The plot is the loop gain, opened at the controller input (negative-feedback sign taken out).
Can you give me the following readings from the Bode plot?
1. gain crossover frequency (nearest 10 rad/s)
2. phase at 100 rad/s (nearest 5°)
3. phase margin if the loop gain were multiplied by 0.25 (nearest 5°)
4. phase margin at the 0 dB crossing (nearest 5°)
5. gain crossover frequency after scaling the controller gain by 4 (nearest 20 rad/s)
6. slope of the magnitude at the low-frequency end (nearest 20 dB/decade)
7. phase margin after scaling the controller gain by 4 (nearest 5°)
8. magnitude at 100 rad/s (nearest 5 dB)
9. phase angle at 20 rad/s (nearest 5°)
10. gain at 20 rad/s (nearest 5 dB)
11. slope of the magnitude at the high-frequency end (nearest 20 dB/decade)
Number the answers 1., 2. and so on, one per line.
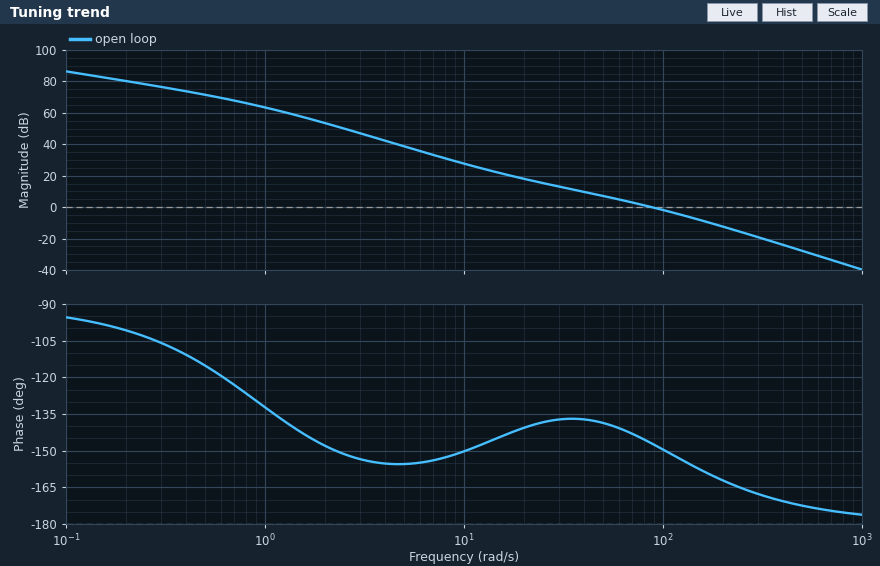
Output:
1. 90 rad/s
2. -150°
3. 45°
4. 35°
5. 200 rad/s
6. -20 dB/decade
7. 20°
8. 0 dB
9. -140°
10. 20 dB
11. -40 dB/decade
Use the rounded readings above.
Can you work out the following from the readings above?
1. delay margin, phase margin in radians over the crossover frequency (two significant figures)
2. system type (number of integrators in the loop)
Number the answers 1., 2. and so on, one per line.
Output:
1. 0.0068 s
2. 1
